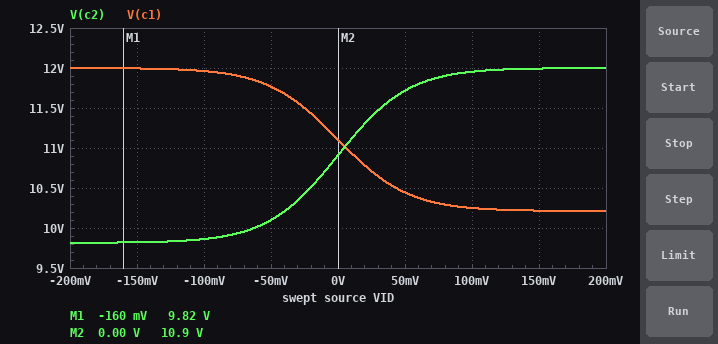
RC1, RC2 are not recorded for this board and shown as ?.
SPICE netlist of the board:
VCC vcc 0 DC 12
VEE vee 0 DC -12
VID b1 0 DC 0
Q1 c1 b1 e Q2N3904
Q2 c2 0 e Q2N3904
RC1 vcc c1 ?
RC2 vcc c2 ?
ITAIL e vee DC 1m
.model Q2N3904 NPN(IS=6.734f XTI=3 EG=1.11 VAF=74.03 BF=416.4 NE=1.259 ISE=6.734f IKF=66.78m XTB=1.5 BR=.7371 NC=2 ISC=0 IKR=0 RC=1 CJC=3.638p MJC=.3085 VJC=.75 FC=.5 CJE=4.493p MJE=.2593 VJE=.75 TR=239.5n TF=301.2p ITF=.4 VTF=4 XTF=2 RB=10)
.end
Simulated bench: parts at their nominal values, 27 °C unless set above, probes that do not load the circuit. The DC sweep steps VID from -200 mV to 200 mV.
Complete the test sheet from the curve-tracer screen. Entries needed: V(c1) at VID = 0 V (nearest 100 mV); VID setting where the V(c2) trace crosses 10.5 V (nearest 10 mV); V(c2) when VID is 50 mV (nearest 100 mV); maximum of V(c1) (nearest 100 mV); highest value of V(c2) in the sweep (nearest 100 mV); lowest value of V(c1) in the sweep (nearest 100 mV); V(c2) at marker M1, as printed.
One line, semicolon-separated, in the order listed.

11.1 V; -20 mV; 11.7 V; 12.0 V; 12.0 V; 10.2 V; 9.82 V
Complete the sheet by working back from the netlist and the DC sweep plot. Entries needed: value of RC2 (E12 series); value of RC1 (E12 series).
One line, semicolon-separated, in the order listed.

2.2 kΩ; 1.8 kΩ
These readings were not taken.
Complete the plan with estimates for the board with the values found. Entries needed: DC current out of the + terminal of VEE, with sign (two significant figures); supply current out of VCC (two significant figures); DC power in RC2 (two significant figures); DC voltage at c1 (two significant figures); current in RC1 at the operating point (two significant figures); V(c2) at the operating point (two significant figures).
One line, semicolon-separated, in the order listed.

-1.0 mA; 990 µA; 540 µW; 11 V; 500 µA; 11 V
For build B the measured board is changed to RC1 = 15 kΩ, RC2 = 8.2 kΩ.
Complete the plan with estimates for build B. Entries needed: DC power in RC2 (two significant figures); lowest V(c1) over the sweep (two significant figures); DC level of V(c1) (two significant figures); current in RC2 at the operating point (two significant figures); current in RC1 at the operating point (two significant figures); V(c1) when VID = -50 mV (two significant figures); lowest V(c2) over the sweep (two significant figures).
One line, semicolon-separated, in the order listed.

2.1 mW; -520 mV; 4.7 V; 510 µA; 490 µA; 10 V; 3.9 V
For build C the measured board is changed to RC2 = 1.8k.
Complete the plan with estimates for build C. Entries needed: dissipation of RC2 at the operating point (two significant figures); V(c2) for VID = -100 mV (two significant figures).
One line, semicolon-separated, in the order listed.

440 µW; 10 V
